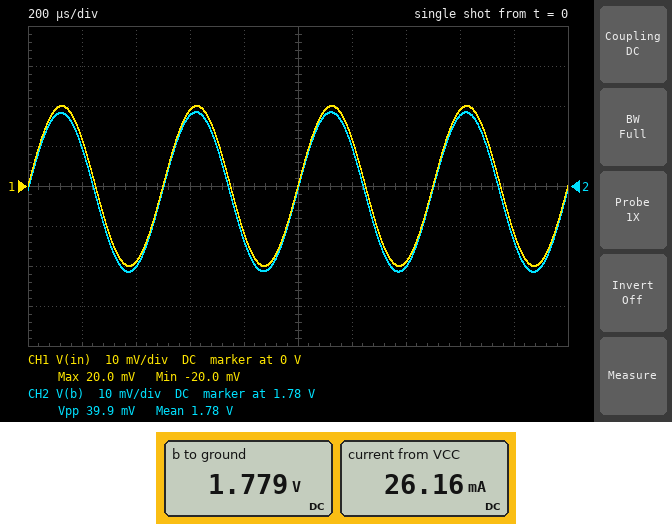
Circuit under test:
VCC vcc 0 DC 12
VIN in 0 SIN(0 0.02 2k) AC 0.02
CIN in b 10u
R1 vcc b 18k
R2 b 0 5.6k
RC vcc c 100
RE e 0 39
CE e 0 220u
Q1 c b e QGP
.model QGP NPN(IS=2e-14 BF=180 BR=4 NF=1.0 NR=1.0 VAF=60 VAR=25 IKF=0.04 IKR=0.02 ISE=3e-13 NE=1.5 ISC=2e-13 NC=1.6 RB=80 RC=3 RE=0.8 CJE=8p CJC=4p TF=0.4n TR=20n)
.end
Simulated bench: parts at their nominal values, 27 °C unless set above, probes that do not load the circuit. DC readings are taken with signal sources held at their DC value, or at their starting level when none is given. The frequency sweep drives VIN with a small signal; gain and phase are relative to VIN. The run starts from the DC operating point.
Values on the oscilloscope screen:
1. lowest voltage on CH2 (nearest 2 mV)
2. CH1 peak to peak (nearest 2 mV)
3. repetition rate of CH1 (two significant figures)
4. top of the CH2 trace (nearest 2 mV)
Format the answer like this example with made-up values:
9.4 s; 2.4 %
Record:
1.758 V; 40 mV; 2.0 kHz; 1.798 V
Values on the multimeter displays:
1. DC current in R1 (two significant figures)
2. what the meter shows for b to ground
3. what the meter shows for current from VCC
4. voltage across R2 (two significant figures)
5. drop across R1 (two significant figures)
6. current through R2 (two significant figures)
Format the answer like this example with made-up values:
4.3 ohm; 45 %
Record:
570 µA; 1.779 V; 26.16 mA; 1.8 V; 10 V; 320 µA
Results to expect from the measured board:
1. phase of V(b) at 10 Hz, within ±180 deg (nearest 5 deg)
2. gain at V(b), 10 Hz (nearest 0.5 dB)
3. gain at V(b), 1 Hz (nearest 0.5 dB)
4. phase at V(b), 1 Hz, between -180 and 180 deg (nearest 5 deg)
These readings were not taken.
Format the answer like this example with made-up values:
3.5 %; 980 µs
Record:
35 deg; -3.5 dB; -19.0 dB; 80 deg
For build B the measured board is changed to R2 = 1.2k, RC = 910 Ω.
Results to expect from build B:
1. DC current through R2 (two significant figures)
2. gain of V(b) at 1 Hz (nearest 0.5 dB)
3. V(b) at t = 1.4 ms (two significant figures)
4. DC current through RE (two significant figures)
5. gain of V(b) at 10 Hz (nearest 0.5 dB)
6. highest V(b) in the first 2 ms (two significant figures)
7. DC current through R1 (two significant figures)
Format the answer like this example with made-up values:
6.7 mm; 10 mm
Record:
610 µA; -24.5 dB; 710 mV; 2.0 mA; -6.0 dB; 750 mV; 630 µA
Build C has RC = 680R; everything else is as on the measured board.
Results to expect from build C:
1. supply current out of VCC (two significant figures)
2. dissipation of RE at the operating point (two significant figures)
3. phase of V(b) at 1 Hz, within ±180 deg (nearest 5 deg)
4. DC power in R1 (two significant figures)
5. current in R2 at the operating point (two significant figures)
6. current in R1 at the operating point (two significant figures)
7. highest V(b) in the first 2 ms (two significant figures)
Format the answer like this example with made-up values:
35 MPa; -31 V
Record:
17 mA; 11 mW; 90 deg; 6.2 mW; 250 µA; 590 µA; 1.4 V
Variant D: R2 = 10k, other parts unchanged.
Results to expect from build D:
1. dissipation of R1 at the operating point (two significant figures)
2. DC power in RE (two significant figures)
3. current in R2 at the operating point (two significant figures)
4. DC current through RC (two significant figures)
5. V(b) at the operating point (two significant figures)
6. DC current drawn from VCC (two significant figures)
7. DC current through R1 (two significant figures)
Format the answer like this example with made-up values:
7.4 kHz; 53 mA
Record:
5.5 mW; 41 mW; 210 µA; 32 mA; 2.1 V; 33 mA; 550 µA
